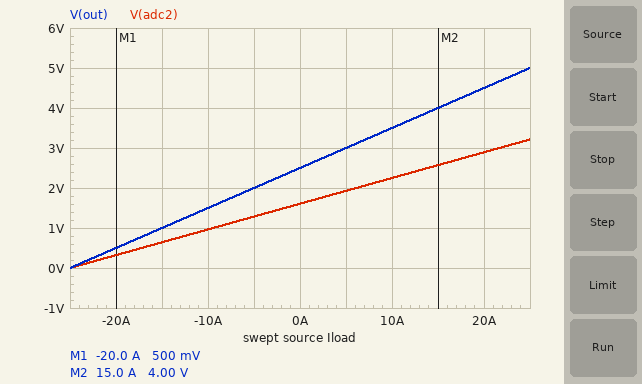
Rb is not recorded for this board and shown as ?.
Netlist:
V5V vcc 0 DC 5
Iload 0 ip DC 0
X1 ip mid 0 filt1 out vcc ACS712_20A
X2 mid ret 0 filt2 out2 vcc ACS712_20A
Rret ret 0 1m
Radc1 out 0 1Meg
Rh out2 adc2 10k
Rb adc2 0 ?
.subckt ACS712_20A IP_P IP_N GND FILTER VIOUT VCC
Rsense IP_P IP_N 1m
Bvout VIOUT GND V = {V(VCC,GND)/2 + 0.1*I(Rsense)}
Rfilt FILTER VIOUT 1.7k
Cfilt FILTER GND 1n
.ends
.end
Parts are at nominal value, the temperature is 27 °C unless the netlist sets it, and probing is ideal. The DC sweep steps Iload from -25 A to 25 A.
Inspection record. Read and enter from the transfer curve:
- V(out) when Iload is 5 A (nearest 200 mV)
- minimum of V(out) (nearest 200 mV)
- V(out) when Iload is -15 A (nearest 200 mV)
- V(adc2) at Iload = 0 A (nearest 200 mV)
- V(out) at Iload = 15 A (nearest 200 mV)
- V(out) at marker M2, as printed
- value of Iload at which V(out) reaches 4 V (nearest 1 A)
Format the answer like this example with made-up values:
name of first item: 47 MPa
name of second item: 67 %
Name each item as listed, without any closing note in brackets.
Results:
V(out) when Iload is 5 A: 3.0 V
minimum of V(out): 0 V
V(out) when Iload is -15 A: 1.0 V
V(adc2) at Iload = 0 A: 1.6 V
V(out) at Iload = 15 A: 4.0 V
V(out) at marker M2, as printed: 4.00 V
value of Iload at which V(out) reaches 4 V: 15 A
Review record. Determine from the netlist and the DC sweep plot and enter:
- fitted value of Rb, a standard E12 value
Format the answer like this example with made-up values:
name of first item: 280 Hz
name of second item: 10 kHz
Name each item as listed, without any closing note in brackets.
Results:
fitted value of Rb, a standard E12 value: 18 kΩ
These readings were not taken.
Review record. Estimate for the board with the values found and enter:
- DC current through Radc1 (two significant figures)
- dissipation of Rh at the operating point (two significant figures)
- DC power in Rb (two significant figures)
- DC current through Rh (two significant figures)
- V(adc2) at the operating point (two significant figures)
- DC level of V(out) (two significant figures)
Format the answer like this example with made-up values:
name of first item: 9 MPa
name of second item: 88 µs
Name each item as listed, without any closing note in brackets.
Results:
DC current through Radc1: 2.5 µA
dissipation of Rh at the operating point: 80 µW
DC power in Rb: 140 µW
DC current through Rh: 89 µA
V(adc2) at the operating point: 1.6 V
DC level of V(out): 2.5 V
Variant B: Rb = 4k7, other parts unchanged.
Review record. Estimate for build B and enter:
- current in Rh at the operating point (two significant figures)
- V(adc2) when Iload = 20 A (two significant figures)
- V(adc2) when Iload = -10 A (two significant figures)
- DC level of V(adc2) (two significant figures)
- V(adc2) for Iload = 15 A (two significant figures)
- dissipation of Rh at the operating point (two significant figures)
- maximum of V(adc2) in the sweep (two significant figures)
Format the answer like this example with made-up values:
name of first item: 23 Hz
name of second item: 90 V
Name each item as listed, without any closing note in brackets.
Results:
current in Rh at the operating point: 170 µA
V(adc2) when Iload = 20 A: 1.4 V
V(adc2) when Iload = -10 A: 480 mV
DC level of V(adc2): 800 mV
V(adc2) for Iload = 15 A: 1.3 V
dissipation of Rh at the operating point: 290 µW
maximum of V(adc2) in the sweep: 1.6 V
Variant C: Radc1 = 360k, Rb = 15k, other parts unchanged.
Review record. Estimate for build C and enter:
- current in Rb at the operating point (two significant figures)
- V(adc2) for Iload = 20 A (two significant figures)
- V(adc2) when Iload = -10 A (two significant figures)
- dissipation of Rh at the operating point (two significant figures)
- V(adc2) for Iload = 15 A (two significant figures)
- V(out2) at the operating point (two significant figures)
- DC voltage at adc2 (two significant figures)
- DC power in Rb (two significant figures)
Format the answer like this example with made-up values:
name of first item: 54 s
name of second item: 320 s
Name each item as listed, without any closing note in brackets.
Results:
current in Rb at the operating point: 100 µA
V(adc2) for Iload = 20 A: 2.7 V
V(adc2) when Iload = -10 A: 900 mV
dissipation of Rh at the operating point: 100 µW
V(adc2) for Iload = 15 A: 2.4 V
V(out2) at the operating point: 2.5 V
DC voltage at adc2: 1.5 V
DC power in Rb: 150 µW
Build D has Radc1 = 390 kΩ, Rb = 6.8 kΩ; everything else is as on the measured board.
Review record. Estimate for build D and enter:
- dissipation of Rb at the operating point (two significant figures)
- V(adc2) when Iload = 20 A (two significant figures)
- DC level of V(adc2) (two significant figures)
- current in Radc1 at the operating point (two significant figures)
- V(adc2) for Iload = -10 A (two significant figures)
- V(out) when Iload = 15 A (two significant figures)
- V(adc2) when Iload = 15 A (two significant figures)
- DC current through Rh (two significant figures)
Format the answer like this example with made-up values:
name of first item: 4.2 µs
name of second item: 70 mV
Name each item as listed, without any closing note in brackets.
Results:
dissipation of Rb at the operating point: 150 µW
V(adc2) when Iload = 20 A: 1.8 V
DC level of V(adc2): 1.0 V
current in Radc1 at the operating point: 6.4 µA
V(adc2) for Iload = -10 A: 610 mV
V(out) when Iload = 15 A: 4.0 V
V(adc2) when Iload = 15 A: 1.6 V
DC current through Rh: 150 µA
